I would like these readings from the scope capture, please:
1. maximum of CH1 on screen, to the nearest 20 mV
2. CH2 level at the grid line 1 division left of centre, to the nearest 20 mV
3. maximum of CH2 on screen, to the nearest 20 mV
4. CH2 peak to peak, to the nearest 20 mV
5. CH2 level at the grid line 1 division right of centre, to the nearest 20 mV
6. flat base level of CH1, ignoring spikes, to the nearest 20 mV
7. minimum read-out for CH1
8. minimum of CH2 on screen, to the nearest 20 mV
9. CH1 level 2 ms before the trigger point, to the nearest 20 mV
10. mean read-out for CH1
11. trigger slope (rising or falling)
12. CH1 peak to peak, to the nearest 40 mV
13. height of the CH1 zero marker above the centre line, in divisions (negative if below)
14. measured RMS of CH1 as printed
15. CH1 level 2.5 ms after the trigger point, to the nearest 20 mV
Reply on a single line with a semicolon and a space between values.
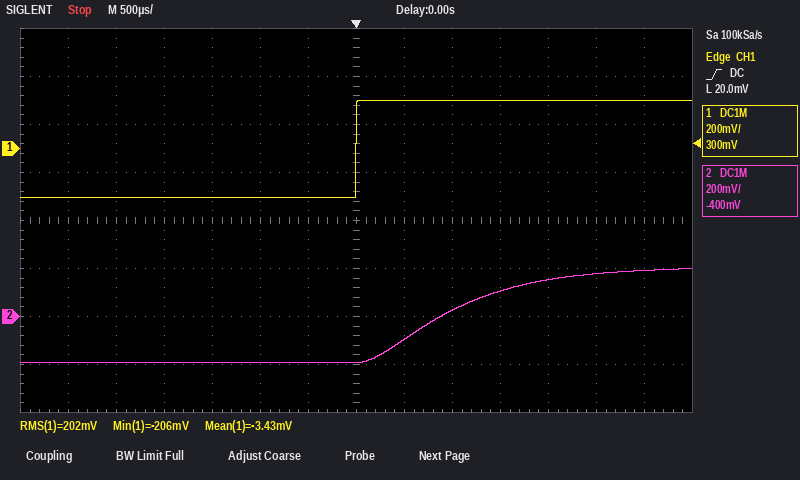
200 mV; -200 mV; 200 mV; 400 mV; -100 mV; -200 mV; -206 mV; -200 mV; -200 mV; -3.43 mV; rising; 400 mV; +1.5 div; 202 mV; 200 mV
